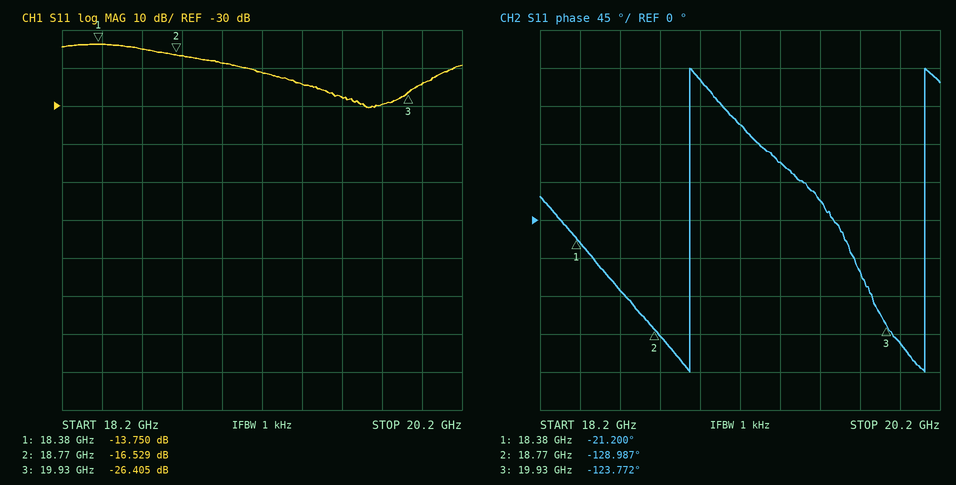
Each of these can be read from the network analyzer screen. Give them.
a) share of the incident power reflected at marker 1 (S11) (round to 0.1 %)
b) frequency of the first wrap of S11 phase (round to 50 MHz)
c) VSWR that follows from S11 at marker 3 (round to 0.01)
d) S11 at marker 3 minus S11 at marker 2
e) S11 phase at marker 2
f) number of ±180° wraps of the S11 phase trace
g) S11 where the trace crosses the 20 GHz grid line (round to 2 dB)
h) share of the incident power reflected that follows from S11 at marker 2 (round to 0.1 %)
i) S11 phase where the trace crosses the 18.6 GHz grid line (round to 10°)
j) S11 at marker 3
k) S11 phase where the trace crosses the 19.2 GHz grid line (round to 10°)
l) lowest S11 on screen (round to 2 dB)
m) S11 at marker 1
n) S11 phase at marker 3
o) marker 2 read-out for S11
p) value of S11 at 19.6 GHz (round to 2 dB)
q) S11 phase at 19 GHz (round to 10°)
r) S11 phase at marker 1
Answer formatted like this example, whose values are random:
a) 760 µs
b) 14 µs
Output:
a) 4.2 %
b) 18.95 GHz
c) 1.10
d) -9.876 dB
e) -128.987°
f) 2
g) -24 dB
h) 2.2 %
i) -80°
j) -26.405 dB
k) 110°
l) -30 dB
m) -13.750 dB
n) -123.772°
o) -16.529 dB
p) -28 dB
q) 170°
r) -21.200°
